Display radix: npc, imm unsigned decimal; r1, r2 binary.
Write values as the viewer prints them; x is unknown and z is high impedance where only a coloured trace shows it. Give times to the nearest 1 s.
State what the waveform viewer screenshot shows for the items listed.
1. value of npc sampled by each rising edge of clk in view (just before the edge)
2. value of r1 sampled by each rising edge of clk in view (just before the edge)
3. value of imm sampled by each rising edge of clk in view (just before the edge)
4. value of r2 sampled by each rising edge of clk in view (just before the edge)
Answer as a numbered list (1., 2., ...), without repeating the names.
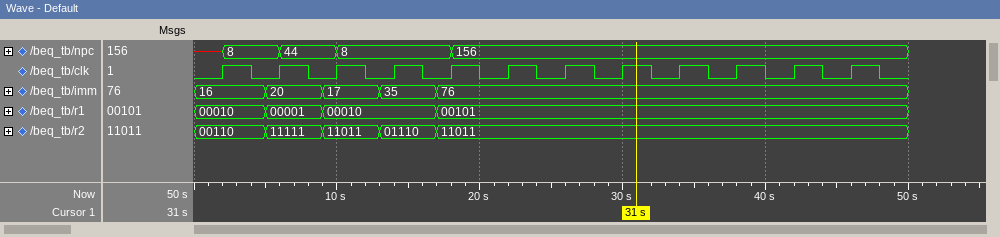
1. x, 8, 44, 8, 8, 156, 156, 156, 156, 156, 156, 156
2. 00010, 00001, 00010, 00010, 00101, 00101, 00101, 00101, 00101, 00101, 00101, 00101
3. 16, 20, 17, 35, 76, 76, 76, 76, 76, 76, 76, 76
4. 00110, 11111, 11011, 01110, 11011, 11011, 11011, 11011, 11011, 11011, 11011, 11011
